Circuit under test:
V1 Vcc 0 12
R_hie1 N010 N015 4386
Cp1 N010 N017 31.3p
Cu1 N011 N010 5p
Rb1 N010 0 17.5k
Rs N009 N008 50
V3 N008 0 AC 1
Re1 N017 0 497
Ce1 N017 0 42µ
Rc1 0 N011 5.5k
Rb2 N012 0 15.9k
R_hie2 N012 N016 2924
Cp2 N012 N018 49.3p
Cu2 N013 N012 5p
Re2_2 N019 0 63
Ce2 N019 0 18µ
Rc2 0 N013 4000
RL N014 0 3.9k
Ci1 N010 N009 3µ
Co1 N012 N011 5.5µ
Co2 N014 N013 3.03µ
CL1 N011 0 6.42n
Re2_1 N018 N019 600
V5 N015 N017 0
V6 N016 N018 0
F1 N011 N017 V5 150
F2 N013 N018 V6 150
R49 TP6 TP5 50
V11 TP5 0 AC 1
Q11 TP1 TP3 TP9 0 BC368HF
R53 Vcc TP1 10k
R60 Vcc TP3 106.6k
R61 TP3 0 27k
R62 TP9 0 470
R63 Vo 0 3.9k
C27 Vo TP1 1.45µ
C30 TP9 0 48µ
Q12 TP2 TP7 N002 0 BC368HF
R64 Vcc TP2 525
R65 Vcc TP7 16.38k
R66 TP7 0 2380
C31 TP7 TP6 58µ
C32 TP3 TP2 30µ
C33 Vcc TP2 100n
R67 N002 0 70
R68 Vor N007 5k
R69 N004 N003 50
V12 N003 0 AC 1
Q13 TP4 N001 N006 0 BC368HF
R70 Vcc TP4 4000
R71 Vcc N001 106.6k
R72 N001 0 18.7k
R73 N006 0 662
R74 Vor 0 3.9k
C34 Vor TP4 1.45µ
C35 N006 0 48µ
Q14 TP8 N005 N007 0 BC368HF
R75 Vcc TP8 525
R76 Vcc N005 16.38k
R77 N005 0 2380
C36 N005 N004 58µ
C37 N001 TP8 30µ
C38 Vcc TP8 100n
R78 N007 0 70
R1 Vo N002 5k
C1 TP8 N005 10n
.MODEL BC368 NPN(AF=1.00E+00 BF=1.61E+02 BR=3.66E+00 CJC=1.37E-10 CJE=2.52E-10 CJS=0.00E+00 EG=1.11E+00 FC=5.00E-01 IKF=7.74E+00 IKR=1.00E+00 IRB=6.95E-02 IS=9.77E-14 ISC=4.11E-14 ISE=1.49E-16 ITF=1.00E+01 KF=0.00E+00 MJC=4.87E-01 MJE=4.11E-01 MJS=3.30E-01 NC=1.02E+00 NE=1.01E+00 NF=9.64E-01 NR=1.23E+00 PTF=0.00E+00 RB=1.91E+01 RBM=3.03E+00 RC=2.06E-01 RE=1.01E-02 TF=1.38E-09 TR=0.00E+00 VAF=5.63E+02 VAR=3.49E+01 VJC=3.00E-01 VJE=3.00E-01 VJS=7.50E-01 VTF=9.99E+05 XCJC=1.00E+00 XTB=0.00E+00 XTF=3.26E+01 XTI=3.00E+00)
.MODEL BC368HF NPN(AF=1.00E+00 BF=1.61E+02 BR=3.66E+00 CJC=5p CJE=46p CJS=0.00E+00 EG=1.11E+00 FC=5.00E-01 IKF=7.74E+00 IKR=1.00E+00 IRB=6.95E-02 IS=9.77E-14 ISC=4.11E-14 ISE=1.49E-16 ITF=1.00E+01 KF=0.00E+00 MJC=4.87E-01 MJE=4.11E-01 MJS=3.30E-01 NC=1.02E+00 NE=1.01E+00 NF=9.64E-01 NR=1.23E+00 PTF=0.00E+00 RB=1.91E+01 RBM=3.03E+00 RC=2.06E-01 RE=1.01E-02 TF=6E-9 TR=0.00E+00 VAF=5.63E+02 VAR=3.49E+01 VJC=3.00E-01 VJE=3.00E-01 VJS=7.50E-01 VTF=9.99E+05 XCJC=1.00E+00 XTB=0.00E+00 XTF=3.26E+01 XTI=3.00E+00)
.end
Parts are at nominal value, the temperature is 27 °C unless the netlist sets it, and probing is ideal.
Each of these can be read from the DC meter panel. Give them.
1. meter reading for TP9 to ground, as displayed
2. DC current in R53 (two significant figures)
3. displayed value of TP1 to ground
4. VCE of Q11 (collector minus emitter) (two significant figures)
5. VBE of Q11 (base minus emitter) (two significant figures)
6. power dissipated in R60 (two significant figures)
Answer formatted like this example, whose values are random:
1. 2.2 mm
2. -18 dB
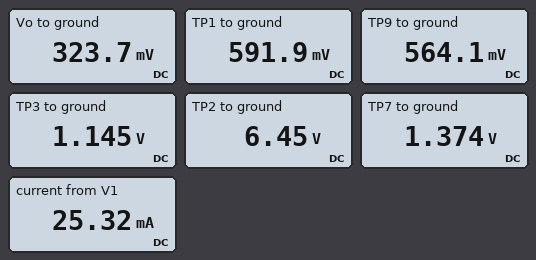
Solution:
1. 564.1 mV
2. 1.1 mA
3. 591.9 mV
4. 28 mV
5. 580 mV
6. 1.1 mW
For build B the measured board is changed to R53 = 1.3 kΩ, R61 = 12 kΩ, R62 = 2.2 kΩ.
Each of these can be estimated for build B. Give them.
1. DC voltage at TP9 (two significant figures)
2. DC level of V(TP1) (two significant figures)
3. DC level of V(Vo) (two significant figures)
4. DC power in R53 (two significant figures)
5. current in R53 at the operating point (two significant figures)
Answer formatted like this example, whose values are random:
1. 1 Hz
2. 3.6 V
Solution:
1. 650 mV
2. 12 V
3. 320 mV
4. 110 µW
5. 290 µA
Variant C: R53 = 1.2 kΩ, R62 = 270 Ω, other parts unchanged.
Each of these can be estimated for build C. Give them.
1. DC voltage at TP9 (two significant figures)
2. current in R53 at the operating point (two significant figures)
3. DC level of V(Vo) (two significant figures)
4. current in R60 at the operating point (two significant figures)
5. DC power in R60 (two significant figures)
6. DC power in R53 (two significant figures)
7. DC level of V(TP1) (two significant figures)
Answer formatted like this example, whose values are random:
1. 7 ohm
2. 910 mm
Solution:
1. 1.2 V
2. 4.3 mA
3. 320 mV
4. 96 µA
5. 980 µW
6. 23 mW
7. 6.8 V
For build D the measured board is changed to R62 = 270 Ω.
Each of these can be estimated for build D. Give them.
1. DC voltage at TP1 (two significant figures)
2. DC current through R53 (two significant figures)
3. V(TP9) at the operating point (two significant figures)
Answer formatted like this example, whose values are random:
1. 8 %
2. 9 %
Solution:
1. 360 mV
2. 1.2 mA
3. 330 mV
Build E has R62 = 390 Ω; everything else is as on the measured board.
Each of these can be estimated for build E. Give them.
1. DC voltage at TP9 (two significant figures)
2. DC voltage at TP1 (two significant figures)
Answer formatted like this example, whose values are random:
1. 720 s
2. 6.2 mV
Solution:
1. 470 mV
2. 500 mV
